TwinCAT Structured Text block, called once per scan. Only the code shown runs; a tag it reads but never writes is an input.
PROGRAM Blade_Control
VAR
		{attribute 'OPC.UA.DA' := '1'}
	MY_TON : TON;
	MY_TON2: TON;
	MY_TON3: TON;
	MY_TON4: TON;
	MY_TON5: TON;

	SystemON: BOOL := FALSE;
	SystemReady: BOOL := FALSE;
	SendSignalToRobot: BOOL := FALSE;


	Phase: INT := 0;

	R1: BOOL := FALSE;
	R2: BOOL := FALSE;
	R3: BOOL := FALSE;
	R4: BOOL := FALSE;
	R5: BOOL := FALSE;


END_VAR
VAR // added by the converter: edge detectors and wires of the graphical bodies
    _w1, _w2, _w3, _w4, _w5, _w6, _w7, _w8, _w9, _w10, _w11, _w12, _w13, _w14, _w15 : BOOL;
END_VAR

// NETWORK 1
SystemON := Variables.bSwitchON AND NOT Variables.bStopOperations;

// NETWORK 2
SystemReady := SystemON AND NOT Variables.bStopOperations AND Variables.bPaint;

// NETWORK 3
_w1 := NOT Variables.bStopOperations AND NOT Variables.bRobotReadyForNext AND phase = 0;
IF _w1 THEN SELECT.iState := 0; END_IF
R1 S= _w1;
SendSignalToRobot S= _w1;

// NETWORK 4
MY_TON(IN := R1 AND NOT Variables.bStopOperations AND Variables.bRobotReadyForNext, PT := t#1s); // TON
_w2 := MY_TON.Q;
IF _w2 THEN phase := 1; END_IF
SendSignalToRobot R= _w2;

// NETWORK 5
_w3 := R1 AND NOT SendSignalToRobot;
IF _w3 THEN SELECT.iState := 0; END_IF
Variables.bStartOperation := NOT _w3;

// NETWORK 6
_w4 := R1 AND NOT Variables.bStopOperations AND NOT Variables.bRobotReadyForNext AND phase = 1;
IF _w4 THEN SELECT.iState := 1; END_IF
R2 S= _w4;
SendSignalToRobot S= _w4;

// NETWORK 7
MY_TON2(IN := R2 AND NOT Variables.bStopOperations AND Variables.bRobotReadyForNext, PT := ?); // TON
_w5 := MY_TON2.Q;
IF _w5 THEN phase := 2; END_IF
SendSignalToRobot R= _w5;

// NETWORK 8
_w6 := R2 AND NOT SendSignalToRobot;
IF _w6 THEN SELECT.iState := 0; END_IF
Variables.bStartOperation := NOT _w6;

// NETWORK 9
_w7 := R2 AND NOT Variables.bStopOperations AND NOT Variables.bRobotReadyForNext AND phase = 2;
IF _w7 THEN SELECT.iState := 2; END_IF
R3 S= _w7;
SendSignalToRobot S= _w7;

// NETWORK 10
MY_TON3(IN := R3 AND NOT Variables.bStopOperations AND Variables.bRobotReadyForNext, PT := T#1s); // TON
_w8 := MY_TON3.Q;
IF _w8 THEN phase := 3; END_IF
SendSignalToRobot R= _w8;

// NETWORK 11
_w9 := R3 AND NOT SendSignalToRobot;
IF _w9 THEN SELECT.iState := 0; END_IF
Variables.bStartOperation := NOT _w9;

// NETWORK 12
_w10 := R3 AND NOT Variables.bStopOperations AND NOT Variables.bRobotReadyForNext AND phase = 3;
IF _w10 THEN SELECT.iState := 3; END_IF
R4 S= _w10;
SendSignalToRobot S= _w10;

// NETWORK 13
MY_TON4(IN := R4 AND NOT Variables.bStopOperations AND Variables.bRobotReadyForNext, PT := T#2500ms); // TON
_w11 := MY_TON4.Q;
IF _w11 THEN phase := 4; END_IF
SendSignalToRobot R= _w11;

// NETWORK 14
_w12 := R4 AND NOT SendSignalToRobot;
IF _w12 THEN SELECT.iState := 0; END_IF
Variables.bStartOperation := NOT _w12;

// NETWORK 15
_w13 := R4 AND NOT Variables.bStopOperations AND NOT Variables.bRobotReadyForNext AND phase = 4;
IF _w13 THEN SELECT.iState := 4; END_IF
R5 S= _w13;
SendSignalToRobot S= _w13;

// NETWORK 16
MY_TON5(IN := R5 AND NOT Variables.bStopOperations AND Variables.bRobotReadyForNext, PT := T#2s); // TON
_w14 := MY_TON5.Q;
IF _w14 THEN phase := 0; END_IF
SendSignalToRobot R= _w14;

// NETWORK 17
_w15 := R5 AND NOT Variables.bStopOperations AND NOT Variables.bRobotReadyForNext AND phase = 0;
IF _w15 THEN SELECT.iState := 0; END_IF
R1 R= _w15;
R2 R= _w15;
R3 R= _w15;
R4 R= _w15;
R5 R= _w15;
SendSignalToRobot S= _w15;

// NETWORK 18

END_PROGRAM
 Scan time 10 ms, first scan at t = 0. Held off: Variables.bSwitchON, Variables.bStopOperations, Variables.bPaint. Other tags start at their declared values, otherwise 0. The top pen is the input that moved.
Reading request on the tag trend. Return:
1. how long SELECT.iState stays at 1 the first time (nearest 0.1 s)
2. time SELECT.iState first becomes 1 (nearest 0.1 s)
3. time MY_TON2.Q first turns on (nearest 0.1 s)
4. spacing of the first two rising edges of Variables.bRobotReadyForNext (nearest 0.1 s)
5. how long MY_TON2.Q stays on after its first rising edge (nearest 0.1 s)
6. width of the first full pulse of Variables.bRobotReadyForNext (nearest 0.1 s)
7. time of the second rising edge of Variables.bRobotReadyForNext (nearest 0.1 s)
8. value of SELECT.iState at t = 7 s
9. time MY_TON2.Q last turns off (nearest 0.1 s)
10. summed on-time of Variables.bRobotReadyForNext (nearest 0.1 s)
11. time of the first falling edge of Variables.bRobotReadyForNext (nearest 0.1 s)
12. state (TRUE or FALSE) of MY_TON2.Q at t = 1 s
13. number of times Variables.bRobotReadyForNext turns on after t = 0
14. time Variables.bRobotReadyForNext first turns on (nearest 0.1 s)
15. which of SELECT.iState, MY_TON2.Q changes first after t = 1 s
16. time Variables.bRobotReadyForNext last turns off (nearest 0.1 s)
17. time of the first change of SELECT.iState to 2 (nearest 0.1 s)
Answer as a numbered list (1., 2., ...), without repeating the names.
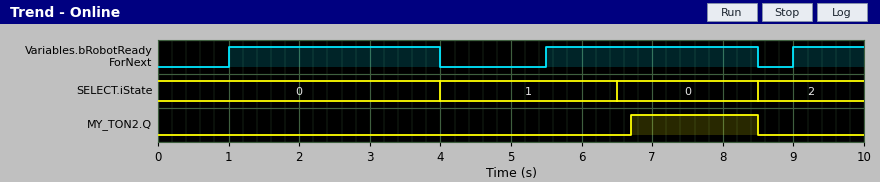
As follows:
1. 2.5 s
2. 4.0 s
3. 6.7 s
4. 4.5 s
5. 1.8 s
6. 3.0 s
7. 5.5 s
8. 0
9. 8.5 s
10. 7.0 s
11. 4.0 s
12. FALSE
13. 3
14. 1.0 s
15. SELECT.iState
16. 8.5 s
17. 8.5 s
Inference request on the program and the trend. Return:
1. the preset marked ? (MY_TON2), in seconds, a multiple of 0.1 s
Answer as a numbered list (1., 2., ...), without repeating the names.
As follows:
1. 1.2 s
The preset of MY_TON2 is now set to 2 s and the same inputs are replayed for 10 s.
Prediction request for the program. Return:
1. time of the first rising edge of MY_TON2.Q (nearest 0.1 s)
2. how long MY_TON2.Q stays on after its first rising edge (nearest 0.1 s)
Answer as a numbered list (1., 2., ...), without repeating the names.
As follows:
1. 7.5 s
2. 1.0 s
